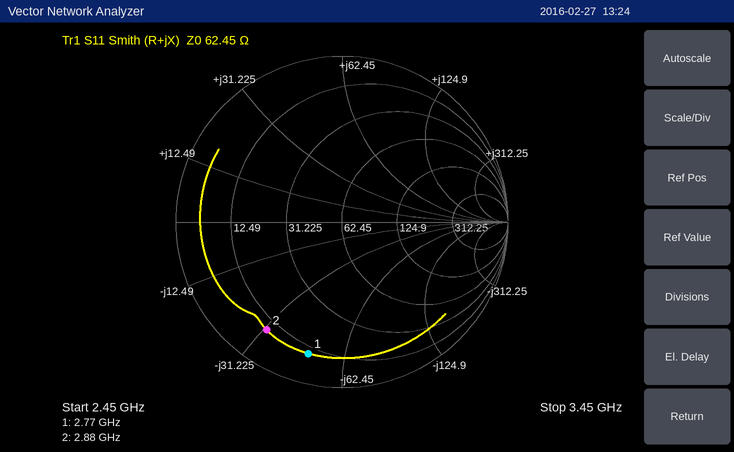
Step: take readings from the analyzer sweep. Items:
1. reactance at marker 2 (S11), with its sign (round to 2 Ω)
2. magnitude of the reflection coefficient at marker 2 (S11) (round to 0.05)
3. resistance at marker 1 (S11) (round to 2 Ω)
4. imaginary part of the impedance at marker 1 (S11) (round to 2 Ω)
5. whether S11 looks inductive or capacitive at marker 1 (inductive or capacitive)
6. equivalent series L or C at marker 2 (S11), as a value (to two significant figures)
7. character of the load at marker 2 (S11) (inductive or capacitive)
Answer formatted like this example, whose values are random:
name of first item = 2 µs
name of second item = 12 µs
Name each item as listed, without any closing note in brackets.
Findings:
reactance at marker 2 (S11), with its sign = -32 Ω
magnitude of the reflection coefficient at marker 2 (S11) = 0.80
resistance at marker 1 (S11) = 10 Ω
imaginary part of the impedance at marker 1 (S11) = -48 Ω
whether S11 looks inductive or capacitive at marker 1 = capacitive
equivalent series L or C at marker 2 (S11), as a value = 1.7 pF
character of the load at marker 2 (S11) = capacitive
